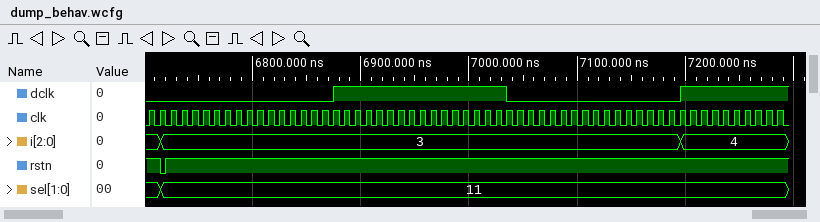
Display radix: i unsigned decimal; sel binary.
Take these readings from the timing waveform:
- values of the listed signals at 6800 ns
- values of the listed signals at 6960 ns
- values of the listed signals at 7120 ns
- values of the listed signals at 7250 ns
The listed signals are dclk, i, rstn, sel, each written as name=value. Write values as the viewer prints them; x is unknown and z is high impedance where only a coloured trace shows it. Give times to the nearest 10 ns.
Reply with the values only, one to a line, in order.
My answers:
dclk=0, i=3, rstn=1, sel=11
dclk=1, i=3, rstn=1, sel=11
dclk=0, i=3, rstn=1, sel=11
dclk=1, i=4, rstn=1, sel=11
